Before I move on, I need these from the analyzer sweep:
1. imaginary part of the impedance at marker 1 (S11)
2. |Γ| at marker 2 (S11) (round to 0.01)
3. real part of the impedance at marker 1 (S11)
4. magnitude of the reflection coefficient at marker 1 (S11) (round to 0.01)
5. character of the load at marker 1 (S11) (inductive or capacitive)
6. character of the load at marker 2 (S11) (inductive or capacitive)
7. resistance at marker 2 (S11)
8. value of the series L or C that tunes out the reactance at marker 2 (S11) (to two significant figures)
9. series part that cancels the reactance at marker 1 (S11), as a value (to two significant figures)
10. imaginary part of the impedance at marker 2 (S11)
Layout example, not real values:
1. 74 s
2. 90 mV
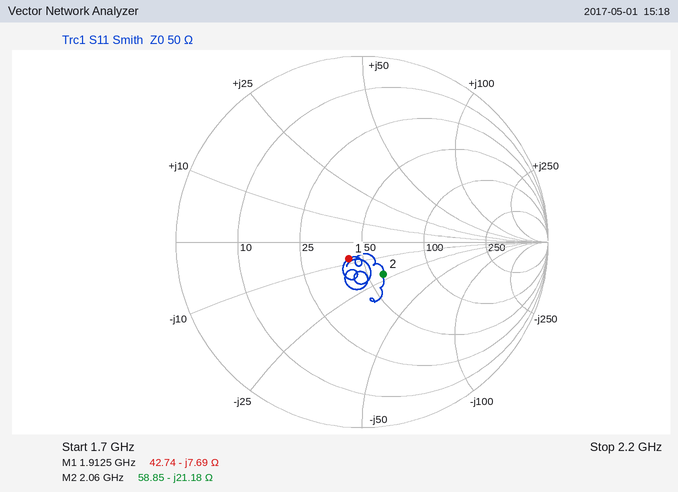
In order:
1. -7.69 Ω
2. 0.21
3. 42.74 Ω
4. 0.11
5. capacitive
6. capacitive
7. 58.85 Ω
8. 1.6 nH
9. 640 pH
10. -21.18 Ω
